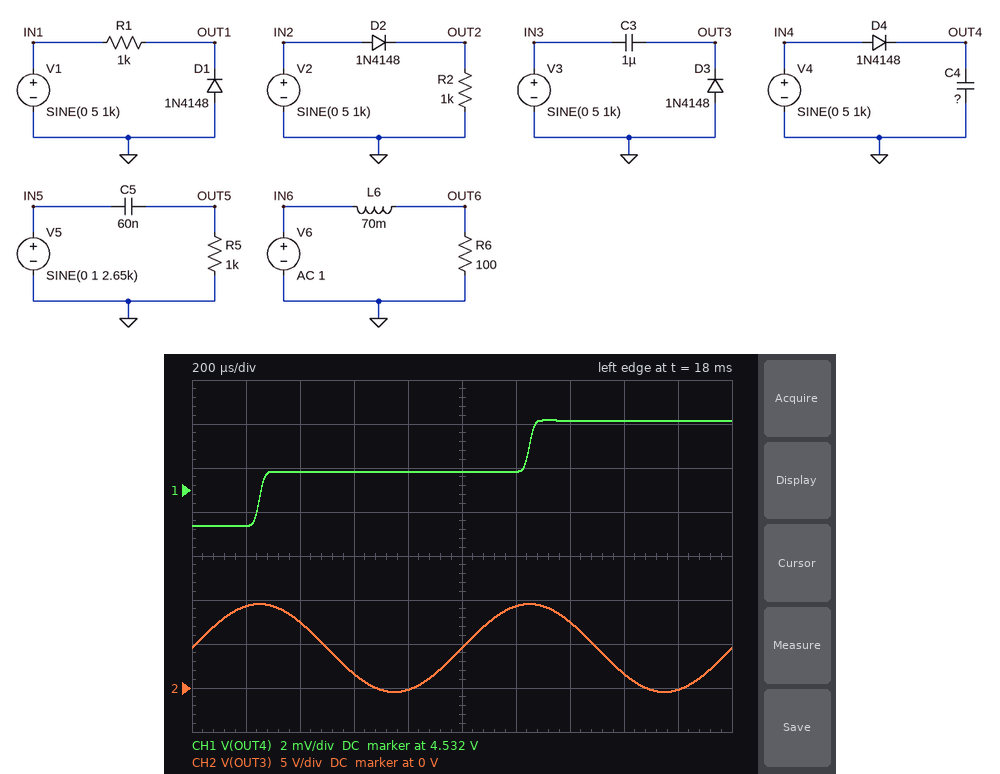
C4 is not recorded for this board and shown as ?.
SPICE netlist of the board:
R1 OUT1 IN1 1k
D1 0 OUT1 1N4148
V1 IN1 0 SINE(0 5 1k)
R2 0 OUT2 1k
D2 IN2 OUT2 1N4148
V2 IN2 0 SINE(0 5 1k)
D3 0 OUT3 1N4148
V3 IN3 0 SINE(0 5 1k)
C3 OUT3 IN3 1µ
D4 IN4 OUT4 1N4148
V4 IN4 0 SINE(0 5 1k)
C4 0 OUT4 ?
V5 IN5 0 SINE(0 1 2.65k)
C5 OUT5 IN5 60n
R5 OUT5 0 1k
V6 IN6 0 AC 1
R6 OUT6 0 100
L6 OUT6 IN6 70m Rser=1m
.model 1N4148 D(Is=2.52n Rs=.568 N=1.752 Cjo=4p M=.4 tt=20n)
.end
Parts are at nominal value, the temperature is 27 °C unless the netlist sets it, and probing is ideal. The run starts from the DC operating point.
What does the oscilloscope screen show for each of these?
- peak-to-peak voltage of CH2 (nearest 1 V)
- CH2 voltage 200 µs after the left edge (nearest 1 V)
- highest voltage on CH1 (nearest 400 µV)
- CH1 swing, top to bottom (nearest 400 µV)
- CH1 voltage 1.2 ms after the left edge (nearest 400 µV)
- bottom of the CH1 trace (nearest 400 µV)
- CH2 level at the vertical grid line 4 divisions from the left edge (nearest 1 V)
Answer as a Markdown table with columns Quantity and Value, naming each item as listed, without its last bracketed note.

| Quantity | Value |
|---|---|
| peak-to-peak voltage of CH2 | 10 V |
| CH2 voltage 200 µs after the left edge | 9 V |
| highest voltage on CH1 | 4.5352 V |
| CH1 swing, top to bottom | 4.8 mV |
| CH1 voltage 1.2 ms after the left edge | 4.5328 V |
| bottom of the CH1 trace | 4.5304 V |
| CH2 level at the vertical grid line 4 divisions from the left edge | 0 V |
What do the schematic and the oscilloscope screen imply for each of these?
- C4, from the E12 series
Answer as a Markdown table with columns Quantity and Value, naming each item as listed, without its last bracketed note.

| Quantity | Value |
|---|---|
| C4, from the E12 series | 1.2 µF |
